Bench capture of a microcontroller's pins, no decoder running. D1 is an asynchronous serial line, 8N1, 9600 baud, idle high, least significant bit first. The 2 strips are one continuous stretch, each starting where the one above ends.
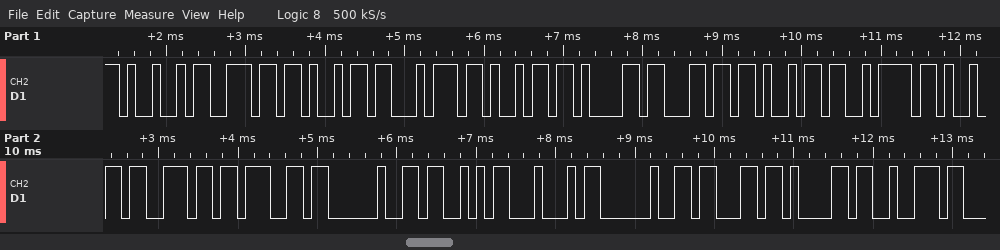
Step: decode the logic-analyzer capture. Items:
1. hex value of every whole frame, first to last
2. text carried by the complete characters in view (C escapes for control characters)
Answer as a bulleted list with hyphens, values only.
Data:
- 0x49 0x6E 0x69 0x74 0x69 0x61 0x6C 0x69 0x7A 0x69 0x6E 0x67 0x20 0x53 0x44 0x20 0x63 0x61 0x72
- "Initializing SD car"
